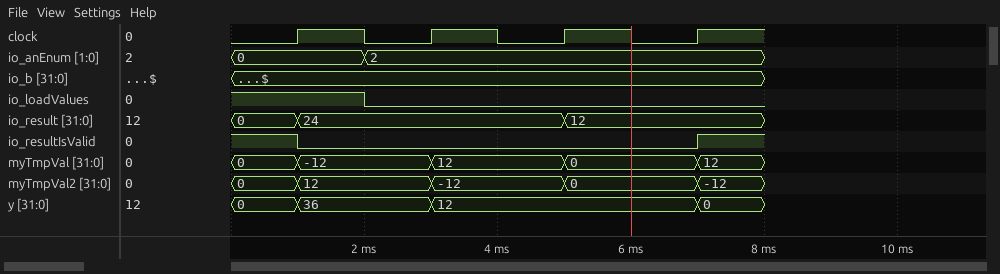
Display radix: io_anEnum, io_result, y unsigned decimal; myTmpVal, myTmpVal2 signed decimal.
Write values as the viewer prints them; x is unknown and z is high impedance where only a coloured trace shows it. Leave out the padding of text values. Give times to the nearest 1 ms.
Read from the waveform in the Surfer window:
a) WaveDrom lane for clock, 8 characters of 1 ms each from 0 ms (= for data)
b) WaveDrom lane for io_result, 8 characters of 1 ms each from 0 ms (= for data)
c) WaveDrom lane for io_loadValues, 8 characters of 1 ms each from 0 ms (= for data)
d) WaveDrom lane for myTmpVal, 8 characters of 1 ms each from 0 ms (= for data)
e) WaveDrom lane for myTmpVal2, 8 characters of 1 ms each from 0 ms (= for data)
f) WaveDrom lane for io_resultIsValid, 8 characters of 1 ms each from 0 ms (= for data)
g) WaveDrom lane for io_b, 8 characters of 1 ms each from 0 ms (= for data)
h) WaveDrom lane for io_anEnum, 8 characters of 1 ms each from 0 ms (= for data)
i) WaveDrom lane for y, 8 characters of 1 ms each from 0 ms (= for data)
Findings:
{name: 'clock', wave: '01010101'}
{name: 'io_result', wave: '==...=..', data: '0 24 12'}
{name: 'io_loadValues', wave: '1.0.....'}
{name: 'myTmpVal', wave: '==.=.=.=', data: '0 -12 12 0 12'}
{name: 'myTmpVal2', wave: '==.=.=.=', data: '0 12 -12 0 -12'}
{name: 'io_resultIsValid', wave: '10.....1'}
{name: 'io_b', wave: '=.......', data: '$'}
{name: 'io_anEnum', wave: '=.=.....', data: '0 2'}
{name: 'y', wave: '==.=...=', data: '0 36 12 0'}
